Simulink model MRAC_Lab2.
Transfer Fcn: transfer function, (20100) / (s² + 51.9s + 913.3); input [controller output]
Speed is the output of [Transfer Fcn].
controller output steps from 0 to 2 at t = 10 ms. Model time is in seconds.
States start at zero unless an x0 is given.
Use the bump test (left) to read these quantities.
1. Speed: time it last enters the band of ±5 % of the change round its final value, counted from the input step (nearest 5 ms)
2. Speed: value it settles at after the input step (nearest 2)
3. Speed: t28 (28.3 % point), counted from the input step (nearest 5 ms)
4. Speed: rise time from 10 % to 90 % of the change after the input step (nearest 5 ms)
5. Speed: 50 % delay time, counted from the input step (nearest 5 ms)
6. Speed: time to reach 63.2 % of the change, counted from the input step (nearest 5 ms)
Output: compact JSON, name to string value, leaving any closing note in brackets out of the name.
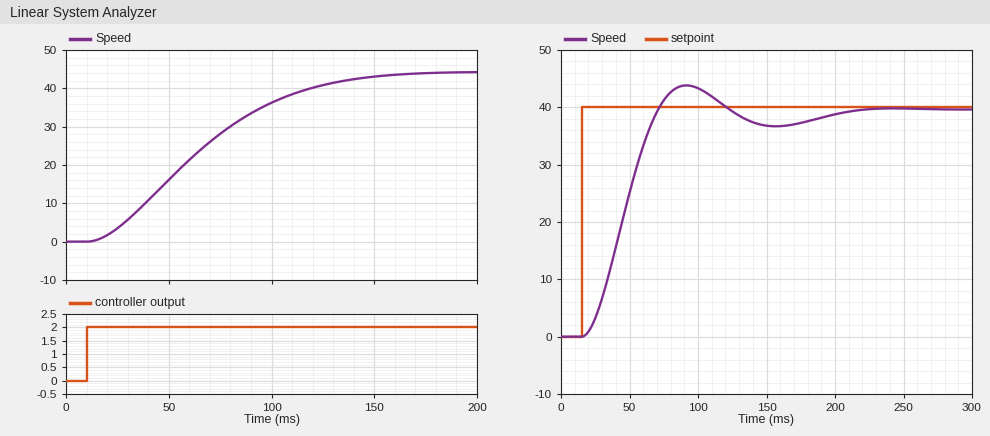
{"Speed: time it last enters the band of ±5 % of the change round its final value, counted from the input step": "125 ms", "Speed: value it settles at after the input step": "44", "Speed: t28 (28.3 % point), counted from the input step": "35 ms", "Speed: rise time from 10 % to 90 % of the change after the input step": "90 ms", "Speed: 50 % delay time, counted from the input step": "50 ms", "Speed: time to reach 63.2 % of the change, counted from the input step": "65 ms"}
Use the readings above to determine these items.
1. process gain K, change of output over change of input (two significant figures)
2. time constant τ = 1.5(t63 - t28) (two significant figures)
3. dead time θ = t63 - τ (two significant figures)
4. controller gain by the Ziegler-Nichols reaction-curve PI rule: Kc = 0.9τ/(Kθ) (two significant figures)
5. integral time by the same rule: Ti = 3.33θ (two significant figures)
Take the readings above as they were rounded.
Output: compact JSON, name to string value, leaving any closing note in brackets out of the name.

{"process gain K, change of output over change of input": "22", "time constant τ = 1.5(t63 - t28)": "45 ms", "dead time θ = t63 - τ": "20 ms", "controller gain by the Ziegler-Nichols reaction-curve PI rule: Kc = 0.9τ/(Kθ)": "0.092", "integral time by the same rule: Ti = 3.33θ": "67 ms"}
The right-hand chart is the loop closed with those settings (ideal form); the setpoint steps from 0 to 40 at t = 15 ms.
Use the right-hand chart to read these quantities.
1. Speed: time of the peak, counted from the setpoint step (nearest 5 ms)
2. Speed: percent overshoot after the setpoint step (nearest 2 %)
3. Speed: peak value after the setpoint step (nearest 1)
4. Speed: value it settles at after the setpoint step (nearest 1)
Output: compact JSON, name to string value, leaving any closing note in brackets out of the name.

{"Speed: time of the peak, counted from the setpoint step": "75 ms", "Speed: percent overshoot after the setpoint step": "10 %", "Speed: peak value after the setpoint step": "44", "Speed: value it settles at after the setpoint step": "40"}
